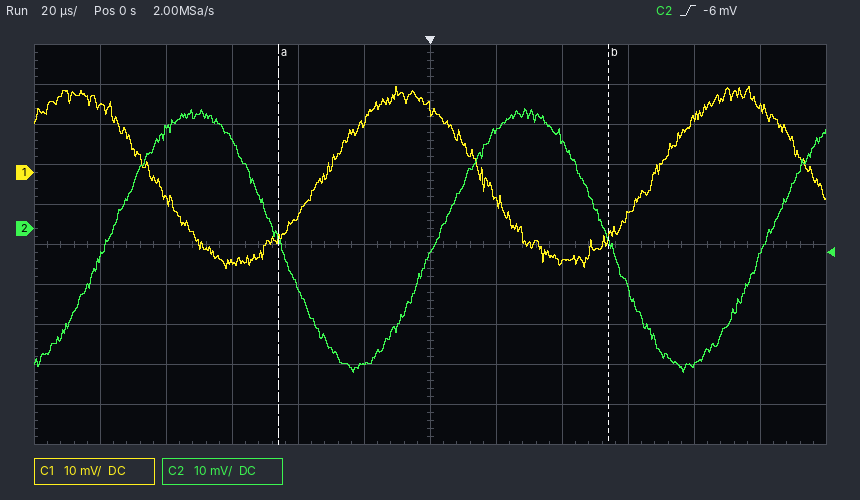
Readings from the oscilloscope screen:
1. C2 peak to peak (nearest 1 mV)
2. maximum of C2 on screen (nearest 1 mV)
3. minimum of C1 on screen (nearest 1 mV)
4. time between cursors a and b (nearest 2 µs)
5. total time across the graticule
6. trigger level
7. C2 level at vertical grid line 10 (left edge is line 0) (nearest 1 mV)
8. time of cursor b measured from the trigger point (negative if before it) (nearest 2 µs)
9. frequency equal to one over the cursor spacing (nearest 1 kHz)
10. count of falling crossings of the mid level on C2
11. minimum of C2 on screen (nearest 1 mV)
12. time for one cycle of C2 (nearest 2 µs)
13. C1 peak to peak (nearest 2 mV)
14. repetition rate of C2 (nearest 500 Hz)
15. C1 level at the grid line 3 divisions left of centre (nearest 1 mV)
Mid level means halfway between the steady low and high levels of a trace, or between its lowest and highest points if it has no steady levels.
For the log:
66 mV
30 mV
-24 mV
100 µs
240 µs
-6 mV
-34 mV
+54 µs
10 kHz
2
-36 mV
100 µs
46 mV
10.0 kHz
-22 mV
